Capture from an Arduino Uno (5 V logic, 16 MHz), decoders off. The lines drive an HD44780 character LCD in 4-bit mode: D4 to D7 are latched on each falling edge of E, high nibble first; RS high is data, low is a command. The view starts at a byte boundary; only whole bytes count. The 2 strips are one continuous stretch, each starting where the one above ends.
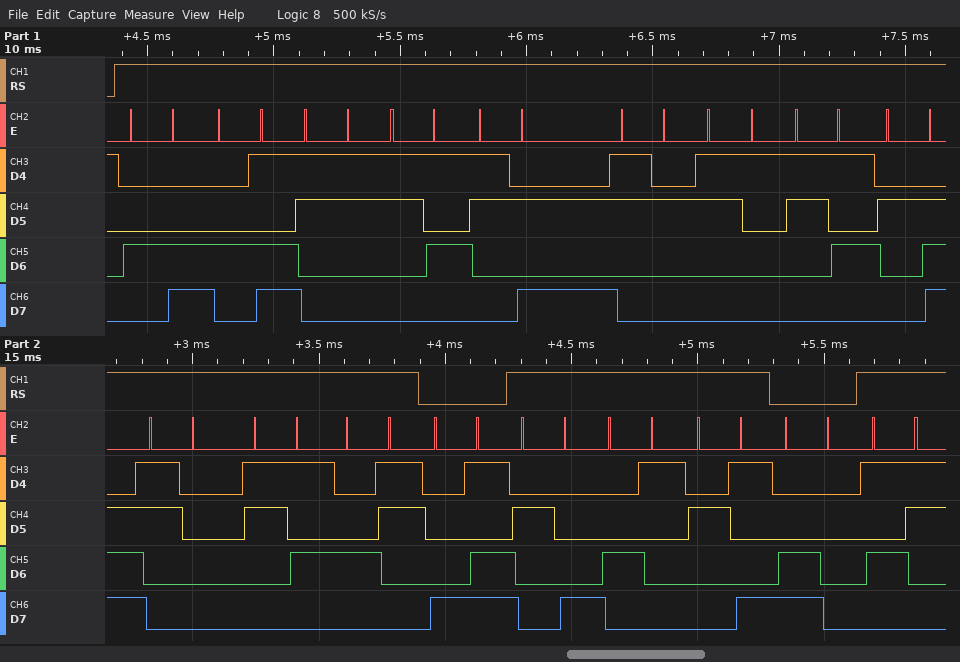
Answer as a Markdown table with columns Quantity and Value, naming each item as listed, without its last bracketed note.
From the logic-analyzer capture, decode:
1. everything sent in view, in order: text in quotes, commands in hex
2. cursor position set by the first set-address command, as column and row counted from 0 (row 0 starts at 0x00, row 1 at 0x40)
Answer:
| Quantity | Value |
|---|---|
| everything sent in view, in order: text in quotes, commands in hex | "LM35:215.05C" 0x8D "(A)" 0xC0 "S" |
| cursor position set by the first set-address command, as column and row counted from 0 | column 13, row 0 |
